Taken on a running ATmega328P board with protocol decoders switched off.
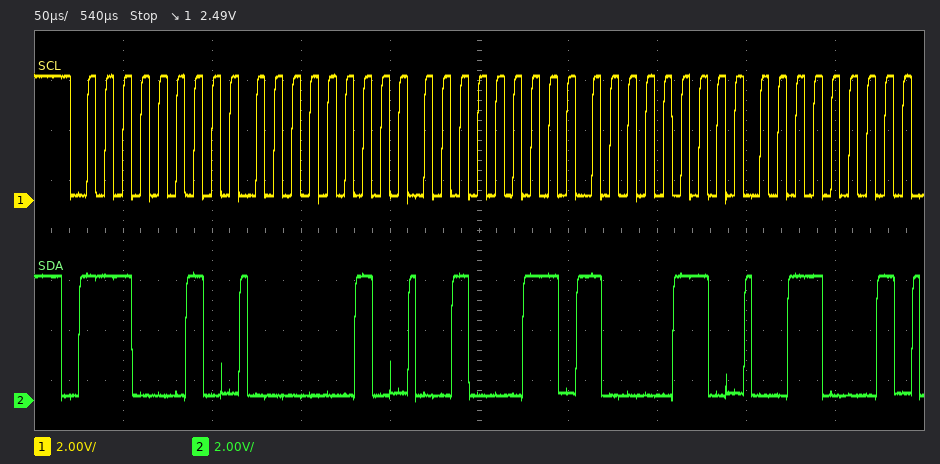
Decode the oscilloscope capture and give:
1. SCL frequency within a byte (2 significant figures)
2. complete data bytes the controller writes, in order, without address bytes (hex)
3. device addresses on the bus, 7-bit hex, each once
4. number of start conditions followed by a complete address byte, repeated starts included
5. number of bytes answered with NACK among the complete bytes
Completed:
100 kHz
02 23 86 31
0x71
1
0
